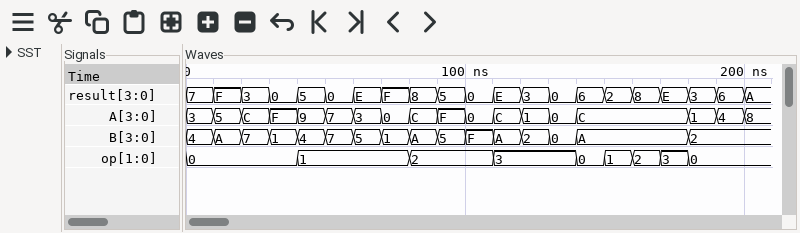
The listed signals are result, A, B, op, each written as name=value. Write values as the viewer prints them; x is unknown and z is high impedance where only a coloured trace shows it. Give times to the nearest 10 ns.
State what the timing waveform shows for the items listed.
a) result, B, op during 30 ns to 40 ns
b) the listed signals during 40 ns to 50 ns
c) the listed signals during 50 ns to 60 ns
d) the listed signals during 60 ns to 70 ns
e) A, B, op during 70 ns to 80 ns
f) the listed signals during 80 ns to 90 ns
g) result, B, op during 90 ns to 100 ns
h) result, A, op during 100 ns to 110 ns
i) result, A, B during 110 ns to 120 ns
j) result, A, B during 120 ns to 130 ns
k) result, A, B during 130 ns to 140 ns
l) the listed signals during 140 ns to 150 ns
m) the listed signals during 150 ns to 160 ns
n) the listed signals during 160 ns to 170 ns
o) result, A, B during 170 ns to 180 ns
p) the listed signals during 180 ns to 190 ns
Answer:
result=0, B=1, op=0
result=5, A=9, B=4, op=1
result=0, A=7, B=7, op=1
result=E, A=3, B=5, op=1
A=0, B=1, op=1
result=8, A=C, B=A, op=2
result=5, B=5, op=2
result=0, A=0, op=2
result=E, A=C, B=A
result=3, A=1, B=2
result=0, A=0, B=0
result=6, A=C, B=A, op=0
result=2, A=C, B=A, op=1
result=8, A=C, B=A, op=2
result=E, A=C, B=A
result=3, A=1, B=2, op=0
